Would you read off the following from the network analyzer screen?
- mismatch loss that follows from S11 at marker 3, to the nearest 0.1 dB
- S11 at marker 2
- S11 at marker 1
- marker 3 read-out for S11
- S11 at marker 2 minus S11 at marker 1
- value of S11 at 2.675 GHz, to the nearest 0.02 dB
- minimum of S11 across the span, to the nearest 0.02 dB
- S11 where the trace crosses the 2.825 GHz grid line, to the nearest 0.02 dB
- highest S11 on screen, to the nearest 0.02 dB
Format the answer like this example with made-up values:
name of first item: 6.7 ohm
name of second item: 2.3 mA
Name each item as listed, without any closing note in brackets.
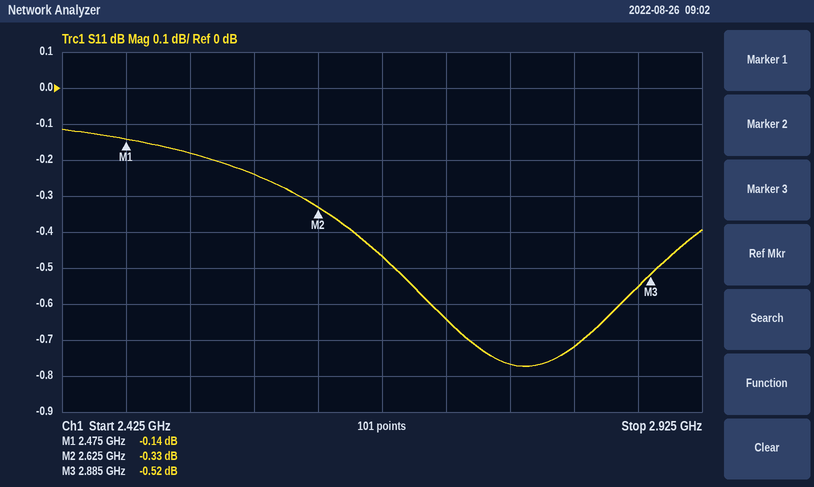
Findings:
mismatch loss that follows from S11 at marker 3, to the nearest 0.1 dB: 9.5 dB
S11 at marker 2: -0.33 dB
S11 at marker 1: -0.14 dB
marker 3 read-out for S11: -0.52 dB
S11 at marker 2 minus S11 at marker 1: -0.19 dB
value of S11 at 2.675 GHz, to the nearest 0.02 dB: -0.46 dB
minimum of S11 across the span, to the nearest 0.02 dB: -0.78 dB
S11 where the trace crosses the 2.825 GHz grid line, to the nearest 0.02 dB: -0.72 dB
highest S11 on screen, to the nearest 0.02 dB: -0.12 dB
